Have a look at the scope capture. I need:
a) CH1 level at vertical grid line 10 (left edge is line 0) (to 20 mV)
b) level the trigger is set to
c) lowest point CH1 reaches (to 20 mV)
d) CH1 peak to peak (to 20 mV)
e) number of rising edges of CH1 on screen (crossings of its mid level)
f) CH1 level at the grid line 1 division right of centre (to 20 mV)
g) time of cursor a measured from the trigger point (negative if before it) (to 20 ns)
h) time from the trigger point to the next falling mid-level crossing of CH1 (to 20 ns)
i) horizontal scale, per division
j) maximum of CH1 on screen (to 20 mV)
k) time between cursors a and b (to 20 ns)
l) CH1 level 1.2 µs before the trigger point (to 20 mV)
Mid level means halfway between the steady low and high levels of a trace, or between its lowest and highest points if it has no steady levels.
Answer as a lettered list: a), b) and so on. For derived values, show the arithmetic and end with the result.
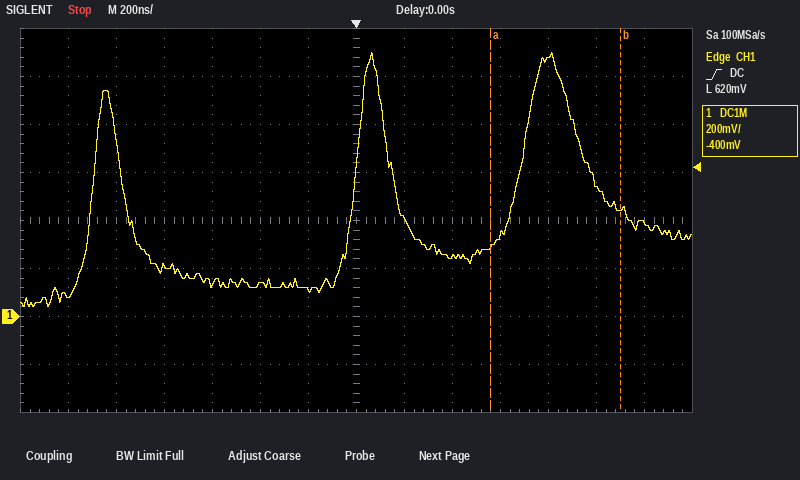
a) 340 mV
b) 620 mV
c) 40 mV
d) 1.10 V − (40 mV) = 1.06 V
e) 3
f) 400 mV
g) +560 ns
h) 160 ns
i) 200 ns
j) 1.10 V
k) 540 ns
l) 80 mV
